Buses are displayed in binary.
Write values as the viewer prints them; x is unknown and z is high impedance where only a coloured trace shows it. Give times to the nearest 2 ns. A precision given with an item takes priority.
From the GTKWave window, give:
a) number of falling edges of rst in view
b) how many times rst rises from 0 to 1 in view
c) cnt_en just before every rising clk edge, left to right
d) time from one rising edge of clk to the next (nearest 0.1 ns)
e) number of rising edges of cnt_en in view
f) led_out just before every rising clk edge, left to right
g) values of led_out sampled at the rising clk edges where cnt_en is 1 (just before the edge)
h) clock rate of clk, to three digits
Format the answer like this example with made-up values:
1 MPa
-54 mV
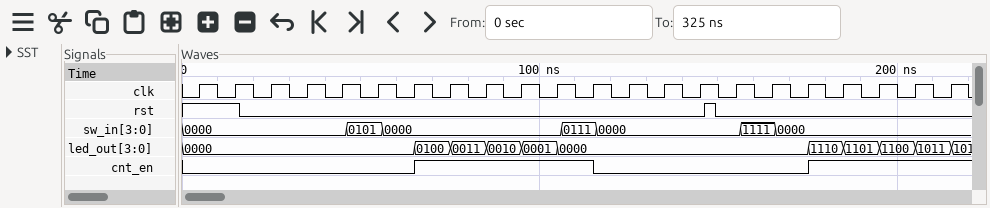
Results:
2
1
0 0 0 0 0 0 0 1 1 1 1 1 0 0 0 0 0 0 1 1 1 1
10 ns
2
0000, 0000, 0000, 0000, 0000, 0000, 0000, 0100, 0011, 0010, 0001, 0000, 0000, 0000, 0000, 0000, 0000, 0000, 1110, 1101, 1100, 1011
0100, 0011, 0010, 0001, 0000, 1110, 1101, 1100, 1011
100 MHz
